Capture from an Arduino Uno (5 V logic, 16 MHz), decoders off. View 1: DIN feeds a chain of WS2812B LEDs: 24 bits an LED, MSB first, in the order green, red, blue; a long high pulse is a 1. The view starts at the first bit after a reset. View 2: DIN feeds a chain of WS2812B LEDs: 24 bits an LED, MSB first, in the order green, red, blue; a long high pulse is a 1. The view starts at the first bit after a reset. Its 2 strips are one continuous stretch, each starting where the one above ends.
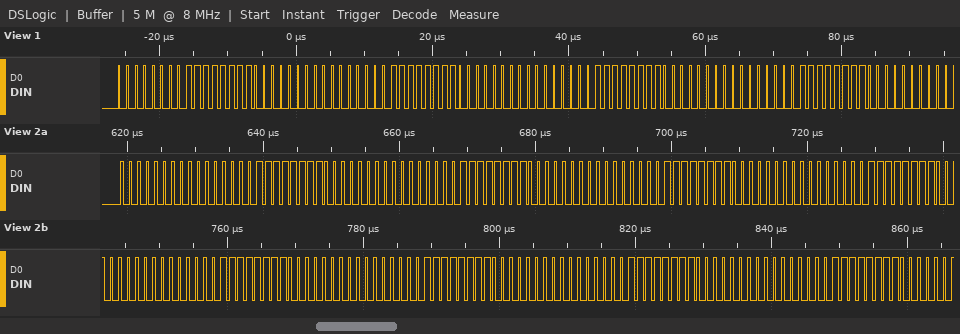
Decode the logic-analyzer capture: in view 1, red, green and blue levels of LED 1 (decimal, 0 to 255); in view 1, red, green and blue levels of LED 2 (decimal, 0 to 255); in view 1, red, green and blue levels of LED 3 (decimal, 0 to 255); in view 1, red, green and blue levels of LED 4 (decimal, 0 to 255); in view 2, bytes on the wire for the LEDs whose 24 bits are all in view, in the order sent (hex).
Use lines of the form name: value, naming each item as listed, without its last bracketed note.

in view 1, red, green and blue levels of LED 1: 255, 0, 0
in view 1, red, green and blue levels of LED 2: 255, 0, 0
in view 1, red, green and blue levels of LED 3: 255, 0, 0
in view 1, red, green and blue levels of LED 4: 255, 0, 0
in view 2, bytes on the wire for the LEDs whose 24 bits are all in view, in the order sent: 00 00 FF 00 00 FF 00 00 FF 00 00 FF 00 00 FF 00 00 FF 00 00 FF 00 00 FF
